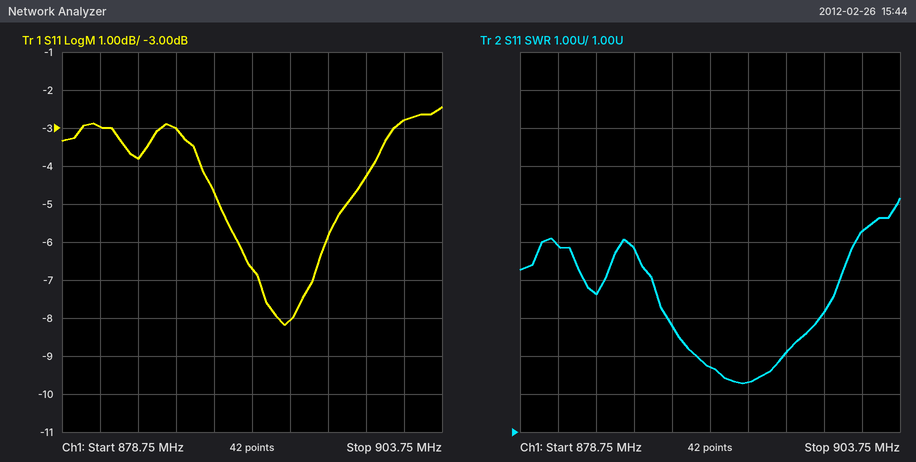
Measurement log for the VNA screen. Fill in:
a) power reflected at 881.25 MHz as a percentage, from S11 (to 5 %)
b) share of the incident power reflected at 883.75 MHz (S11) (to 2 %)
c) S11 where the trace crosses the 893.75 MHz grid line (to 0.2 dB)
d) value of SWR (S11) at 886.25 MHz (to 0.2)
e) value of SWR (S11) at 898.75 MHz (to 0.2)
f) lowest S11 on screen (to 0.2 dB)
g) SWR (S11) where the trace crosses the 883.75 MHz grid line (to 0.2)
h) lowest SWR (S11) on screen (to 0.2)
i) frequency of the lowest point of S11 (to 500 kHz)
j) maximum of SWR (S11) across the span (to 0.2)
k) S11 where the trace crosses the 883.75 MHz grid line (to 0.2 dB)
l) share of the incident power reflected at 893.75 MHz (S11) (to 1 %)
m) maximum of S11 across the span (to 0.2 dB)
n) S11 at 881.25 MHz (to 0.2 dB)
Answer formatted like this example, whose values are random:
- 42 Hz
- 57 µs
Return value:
- 50 %
- 42 %
- -8.0 dB
- 5.8
- 4.2
- -8.2 dB
- 4.6
- 2.2
- 893.5 MHz
- 7.2
- -3.8 dB
- 16 %
- -2.4 dB
- -3.0 dB
